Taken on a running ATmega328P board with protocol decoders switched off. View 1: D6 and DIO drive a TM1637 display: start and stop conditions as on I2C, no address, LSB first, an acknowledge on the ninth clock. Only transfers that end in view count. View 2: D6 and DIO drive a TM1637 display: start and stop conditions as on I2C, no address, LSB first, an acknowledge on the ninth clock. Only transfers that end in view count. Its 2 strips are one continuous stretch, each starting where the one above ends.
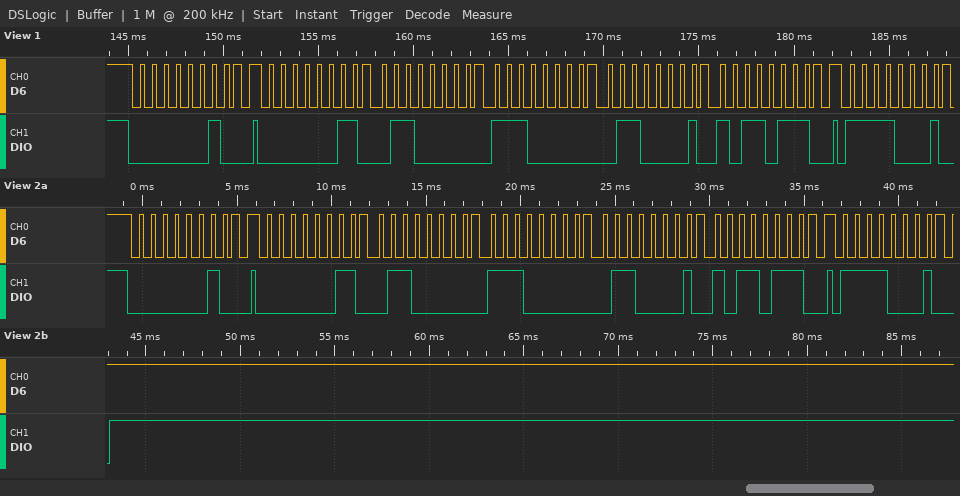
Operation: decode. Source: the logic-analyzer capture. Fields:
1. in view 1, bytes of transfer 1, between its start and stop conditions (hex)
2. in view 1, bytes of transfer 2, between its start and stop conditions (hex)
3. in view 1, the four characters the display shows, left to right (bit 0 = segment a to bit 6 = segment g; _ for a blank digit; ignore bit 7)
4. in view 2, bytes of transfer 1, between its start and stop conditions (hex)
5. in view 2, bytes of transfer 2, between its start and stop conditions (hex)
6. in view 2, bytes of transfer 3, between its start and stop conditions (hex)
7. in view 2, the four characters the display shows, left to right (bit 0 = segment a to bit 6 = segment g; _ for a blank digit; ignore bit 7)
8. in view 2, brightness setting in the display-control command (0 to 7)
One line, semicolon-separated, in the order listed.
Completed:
40; C0 06 07 86 ED; 1715; 40; C0 06 07 86 ED; 8F; 1715; 7
